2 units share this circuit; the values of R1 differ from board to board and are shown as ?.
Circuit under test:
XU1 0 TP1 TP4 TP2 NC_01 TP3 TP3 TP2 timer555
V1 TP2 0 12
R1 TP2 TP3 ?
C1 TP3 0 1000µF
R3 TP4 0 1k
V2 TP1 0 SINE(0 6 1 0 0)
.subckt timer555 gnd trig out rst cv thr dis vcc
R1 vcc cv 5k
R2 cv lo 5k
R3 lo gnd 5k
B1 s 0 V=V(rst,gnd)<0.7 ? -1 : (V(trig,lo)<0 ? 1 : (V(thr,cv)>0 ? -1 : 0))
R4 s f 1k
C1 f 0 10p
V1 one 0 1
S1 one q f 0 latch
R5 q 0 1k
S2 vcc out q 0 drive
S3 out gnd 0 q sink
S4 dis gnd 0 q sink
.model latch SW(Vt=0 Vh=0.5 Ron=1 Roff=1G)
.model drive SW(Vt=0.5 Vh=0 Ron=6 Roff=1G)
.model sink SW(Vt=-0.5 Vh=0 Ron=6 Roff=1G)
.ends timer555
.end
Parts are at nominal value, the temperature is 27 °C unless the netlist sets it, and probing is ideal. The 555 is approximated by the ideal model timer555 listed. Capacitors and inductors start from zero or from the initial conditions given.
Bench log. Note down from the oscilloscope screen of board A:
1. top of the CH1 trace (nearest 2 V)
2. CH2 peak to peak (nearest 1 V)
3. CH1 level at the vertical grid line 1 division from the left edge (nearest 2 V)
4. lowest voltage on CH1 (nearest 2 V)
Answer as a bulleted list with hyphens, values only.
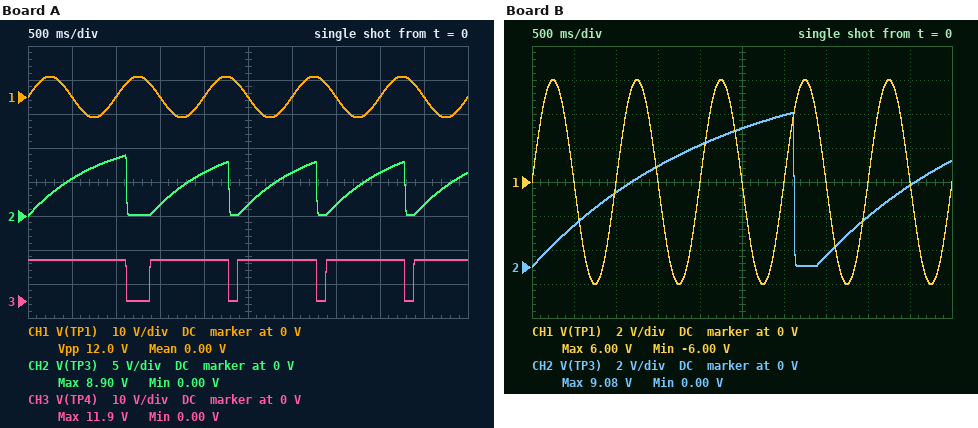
- 6 V
- 9 V
- 0 V
- -6 V
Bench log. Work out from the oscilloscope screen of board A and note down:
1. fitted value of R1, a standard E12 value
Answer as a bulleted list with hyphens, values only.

- 820 Ω
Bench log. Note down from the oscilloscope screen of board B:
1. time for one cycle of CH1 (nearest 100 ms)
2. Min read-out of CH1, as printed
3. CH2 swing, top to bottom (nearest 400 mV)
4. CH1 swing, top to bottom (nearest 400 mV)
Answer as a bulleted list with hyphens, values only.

- 1.0 s
- -6.00 V
- 9.2 V
- 12.0 V
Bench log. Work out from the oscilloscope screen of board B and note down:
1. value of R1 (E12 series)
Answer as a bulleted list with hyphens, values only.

- 2.2 kΩ
